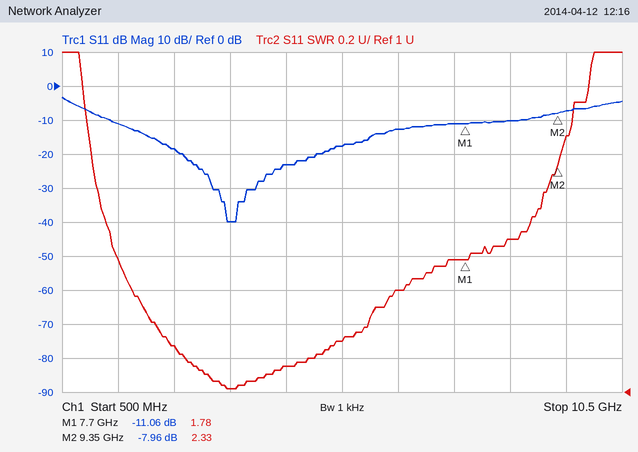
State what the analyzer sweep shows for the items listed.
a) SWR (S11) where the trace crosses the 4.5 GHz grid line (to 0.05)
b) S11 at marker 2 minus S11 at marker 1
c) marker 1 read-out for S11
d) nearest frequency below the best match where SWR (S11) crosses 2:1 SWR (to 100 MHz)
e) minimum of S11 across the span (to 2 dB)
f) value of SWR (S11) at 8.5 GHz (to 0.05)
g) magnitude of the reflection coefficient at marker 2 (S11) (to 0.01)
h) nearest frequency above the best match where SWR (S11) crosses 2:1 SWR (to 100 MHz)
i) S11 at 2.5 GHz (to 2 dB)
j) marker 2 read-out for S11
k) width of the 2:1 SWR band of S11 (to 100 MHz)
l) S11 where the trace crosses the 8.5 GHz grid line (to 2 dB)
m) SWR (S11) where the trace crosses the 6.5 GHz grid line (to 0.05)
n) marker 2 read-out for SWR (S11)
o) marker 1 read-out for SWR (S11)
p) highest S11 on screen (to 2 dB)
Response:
1.15
3.10 dB
-11.06 dB
1.3 GHz
-40 dB
1.90
0.40
8.9 GHz
-18 dB
-7.96 dB
7.6 GHz
-10 dB
1.60
2.33
1.78
-4 dB
